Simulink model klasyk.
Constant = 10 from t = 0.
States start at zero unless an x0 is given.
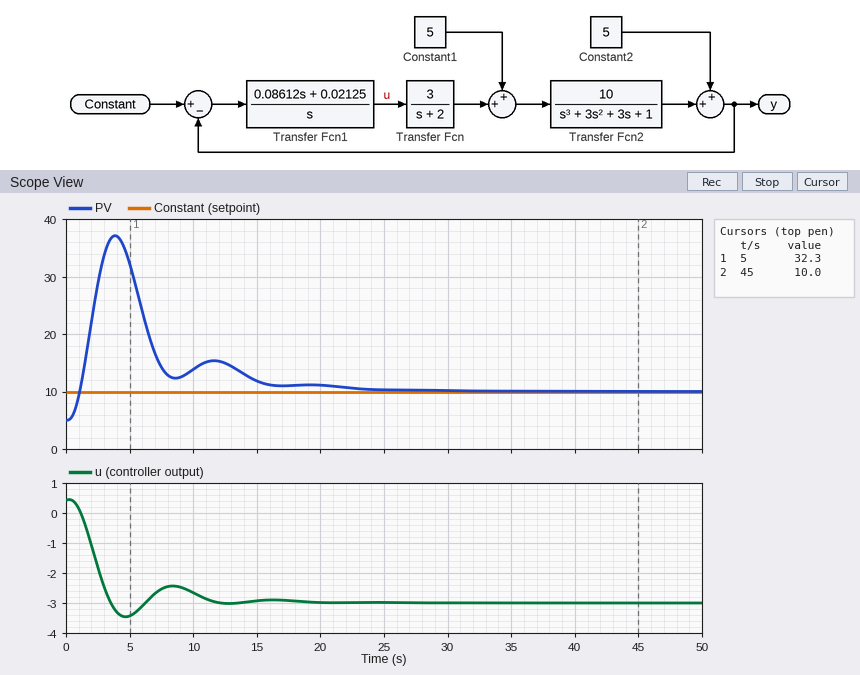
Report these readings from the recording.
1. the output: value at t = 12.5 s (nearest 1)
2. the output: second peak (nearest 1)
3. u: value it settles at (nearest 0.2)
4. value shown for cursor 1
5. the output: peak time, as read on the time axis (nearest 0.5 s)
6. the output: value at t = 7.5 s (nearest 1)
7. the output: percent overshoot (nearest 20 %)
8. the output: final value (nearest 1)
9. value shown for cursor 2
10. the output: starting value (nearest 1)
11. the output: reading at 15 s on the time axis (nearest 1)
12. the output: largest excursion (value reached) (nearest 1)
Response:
15
15
-3.0
32.3
4.0 s
14
540 %
10
10.0
5
12
37
